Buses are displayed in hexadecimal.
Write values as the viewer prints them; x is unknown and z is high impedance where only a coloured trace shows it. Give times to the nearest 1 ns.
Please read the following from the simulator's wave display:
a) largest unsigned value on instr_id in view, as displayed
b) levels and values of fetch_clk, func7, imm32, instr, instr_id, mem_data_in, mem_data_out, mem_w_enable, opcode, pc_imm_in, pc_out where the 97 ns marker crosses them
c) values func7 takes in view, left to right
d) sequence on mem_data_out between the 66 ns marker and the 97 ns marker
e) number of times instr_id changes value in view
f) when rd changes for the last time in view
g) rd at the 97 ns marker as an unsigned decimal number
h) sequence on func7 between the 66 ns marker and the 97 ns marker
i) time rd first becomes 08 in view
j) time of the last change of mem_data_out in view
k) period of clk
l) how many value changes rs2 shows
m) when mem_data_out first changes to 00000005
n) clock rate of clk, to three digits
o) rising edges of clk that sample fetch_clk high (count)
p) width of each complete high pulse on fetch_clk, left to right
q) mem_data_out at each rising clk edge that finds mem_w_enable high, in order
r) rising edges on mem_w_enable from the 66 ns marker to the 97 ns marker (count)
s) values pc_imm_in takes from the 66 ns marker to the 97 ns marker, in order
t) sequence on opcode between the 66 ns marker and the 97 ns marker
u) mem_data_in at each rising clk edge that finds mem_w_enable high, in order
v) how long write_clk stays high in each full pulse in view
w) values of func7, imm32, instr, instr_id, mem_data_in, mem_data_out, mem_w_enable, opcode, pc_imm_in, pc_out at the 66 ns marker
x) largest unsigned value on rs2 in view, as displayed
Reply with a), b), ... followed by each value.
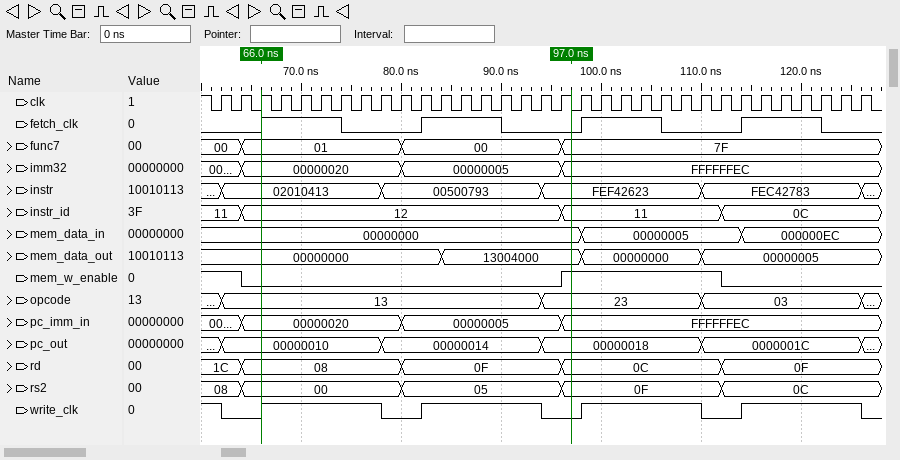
a) 12
b) fetch_clk=0, func7=7F, imm32=FFFFFFEC, instr=FEF42623, instr_id=11, mem_data_in=00000000, mem_data_out=13004000, mem_w_enable=1, opcode=23, pc_imm_in=FFFFFFEC, pc_out=00000018
c) 00, 01, 00, 7F
d) 00000000, 13004000
e) 3
f) 112 ns
g) 12
h) 01, 00, 7F
i) 64 ns
j) 110 ns
k) 2 ns
l) 4
m) 110 ns
n) 500 MHz
o) 16
p) 8 ns, 8 ns, 8 ns, 8 ns
q) 00000000, 00000000, 13004000, 00000000, 00000000, 00000000, 00000000, 00000000, 00000000, 00000005
r) 1
s) 00000020, 00000005, FFFFFFEC
t) 13, 23
u) 00000000, 00000000, 00000000, 00000005, 00000005, 00000005, 00000005, 00000005, 00000005, 00000005
v) 12 ns, 12 ns, 12 ns, 12 ns
w) func7=01, imm32=00000020, instr=02010413, instr_id=12, mem_data_in=00000000, mem_data_out=00000000, mem_w_enable=0, opcode=13, pc_imm_in=00000020, pc_out=00000010
x) 0F
